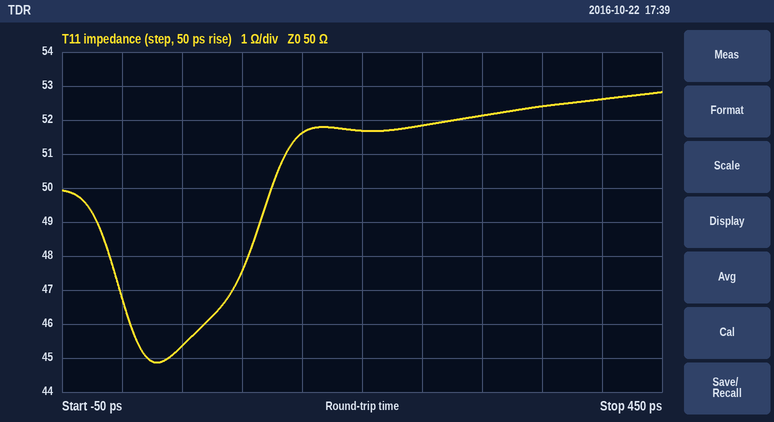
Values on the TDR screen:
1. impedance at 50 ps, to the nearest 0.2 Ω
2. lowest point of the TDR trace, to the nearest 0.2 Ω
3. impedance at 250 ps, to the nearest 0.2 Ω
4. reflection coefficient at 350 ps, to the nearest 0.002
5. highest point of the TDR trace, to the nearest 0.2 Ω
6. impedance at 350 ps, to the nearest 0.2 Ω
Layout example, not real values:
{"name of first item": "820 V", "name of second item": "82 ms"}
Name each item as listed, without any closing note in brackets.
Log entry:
{"impedance at 50 ps, to the nearest 0.2 Ω": "45.4 Ω", "lowest point of the TDR trace, to the nearest 0.2 Ω": "44.8 Ω", "impedance at 250 ps, to the nearest 0.2 Ω": "51.8 Ω", "reflection coefficient at 350 ps, to the nearest 0.002": "+0.024", "highest point of the TDR trace, to the nearest 0.2 Ω": "52.8 Ω", "impedance at 350 ps, to the nearest 0.2 Ω": "52.4 Ω"}
